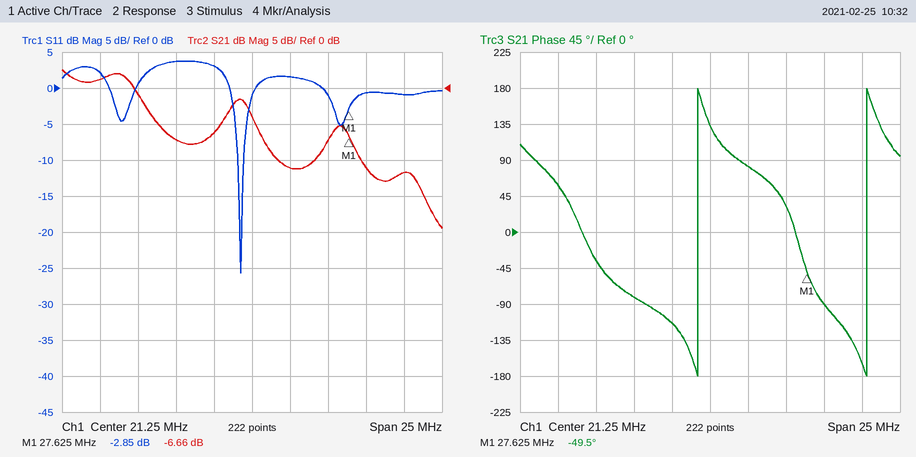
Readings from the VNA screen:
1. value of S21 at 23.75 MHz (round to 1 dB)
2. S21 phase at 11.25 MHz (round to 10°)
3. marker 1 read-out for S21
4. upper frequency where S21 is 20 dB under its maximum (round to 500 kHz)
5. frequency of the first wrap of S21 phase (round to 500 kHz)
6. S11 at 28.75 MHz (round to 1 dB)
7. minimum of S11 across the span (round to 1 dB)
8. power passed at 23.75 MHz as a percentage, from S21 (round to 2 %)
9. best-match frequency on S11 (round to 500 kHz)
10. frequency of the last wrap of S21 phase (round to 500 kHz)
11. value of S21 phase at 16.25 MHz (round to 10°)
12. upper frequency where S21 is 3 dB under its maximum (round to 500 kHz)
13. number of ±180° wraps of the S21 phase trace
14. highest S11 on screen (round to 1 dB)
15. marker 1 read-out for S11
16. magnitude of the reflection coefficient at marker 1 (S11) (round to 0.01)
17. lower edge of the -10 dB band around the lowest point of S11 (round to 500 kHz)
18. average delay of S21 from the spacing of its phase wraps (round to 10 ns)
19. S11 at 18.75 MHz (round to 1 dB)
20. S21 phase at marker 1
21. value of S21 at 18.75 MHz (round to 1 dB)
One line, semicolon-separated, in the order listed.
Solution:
-11 dB; 60°; -6.66 dB; 33.0 MHz; 20.5 MHz; -1 dB; -26 dB; 8 %; 20.5 MHz; 31.5 MHz; -80°; 13.5 MHz; 2; 4 dB; -2.85 dB; 0.72; 20.5 MHz; 90 ns; 3 dB; -49.5°; -6 dB
